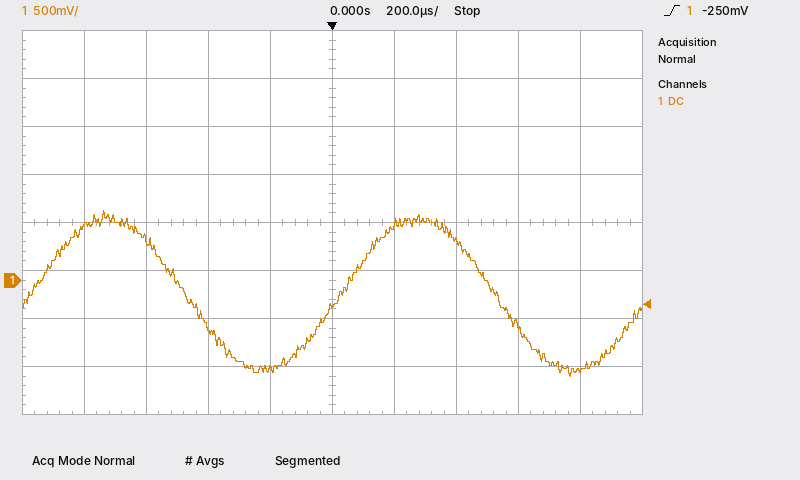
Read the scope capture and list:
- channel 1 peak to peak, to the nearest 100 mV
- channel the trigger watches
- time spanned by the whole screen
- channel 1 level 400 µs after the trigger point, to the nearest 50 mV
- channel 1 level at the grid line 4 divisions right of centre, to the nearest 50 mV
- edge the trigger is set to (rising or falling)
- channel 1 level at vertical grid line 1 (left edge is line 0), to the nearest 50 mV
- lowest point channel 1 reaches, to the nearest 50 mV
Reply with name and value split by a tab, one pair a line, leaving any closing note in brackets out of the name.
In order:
channel 1 peak to peak, to the nearest 100 mV	1.70 V
channel the trigger watches	channel 1
time spanned by the whole screen	2 ms
channel 1 level 400 µs after the trigger point, to the nearest 50 mV	400 mV
channel 1 level at the grid line 4 divisions right of centre, to the nearest 50 mV	-950 mV
edge the trigger is set to	rising
channel 1 level at vertical grid line 1 (left edge is line 0), to the nearest 50 mV	550 mV
lowest point channel 1 reaches, to the nearest 50 mV	-1.00 V
